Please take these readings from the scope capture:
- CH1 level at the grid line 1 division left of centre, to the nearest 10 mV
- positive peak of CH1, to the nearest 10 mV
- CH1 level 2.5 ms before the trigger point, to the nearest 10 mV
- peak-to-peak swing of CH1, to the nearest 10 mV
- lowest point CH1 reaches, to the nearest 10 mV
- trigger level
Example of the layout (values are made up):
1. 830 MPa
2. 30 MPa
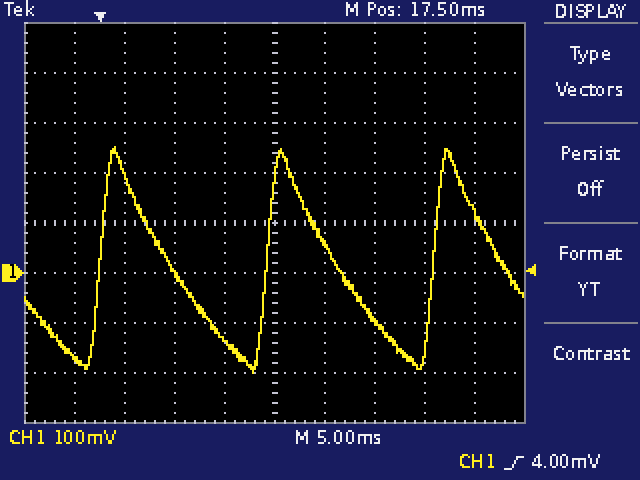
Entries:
1. -140 mV
2. 250 mV
3. -170 mV
4. 450 mV
5. -200 mV
6. 4.00 mV
